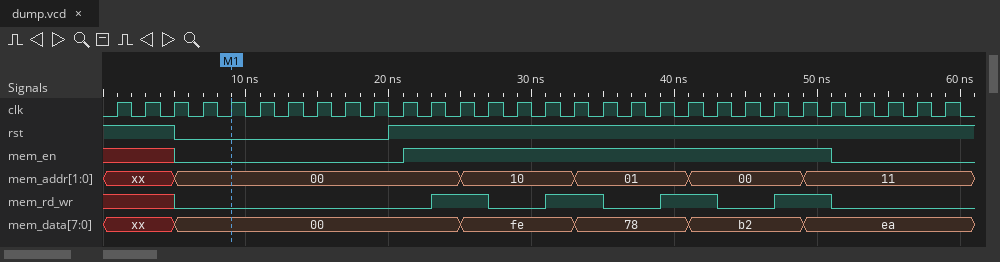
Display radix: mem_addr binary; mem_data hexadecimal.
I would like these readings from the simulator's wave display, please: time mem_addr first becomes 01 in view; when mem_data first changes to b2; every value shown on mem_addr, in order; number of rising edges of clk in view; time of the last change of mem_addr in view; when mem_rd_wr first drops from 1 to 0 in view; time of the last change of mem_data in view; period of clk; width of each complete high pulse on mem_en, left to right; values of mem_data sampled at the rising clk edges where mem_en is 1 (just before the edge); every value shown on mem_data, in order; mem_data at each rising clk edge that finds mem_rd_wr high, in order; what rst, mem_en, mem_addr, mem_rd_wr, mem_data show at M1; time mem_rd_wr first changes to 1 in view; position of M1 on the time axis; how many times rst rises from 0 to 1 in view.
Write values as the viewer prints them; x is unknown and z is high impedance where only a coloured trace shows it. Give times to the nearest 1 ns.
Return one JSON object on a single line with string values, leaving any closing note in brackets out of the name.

{"time mem_addr first becomes 01 in view": "33 ns", "when mem_data first changes to b2": "41 ns", "every value shown on mem_addr, in order": "xx, 00, 10, 01, 00, 11", "number of rising edges of clk in view": "30", "time of the last change of mem_addr in view": "49 ns", "when mem_rd_wr first drops from 1 to 0 in view": "27 ns", "time of the last change of mem_data in view": "49 ns", "period of clk": "2 ns", "width of each complete high pulse on mem_en, left to right": "30 ns", "values of mem_data sampled at the rising clk edges where mem_en is 1": "00, 00, fe, fe, fe, fe, 78, 78, 78, 78, b2, b2, b2, b2, ea", "every value shown on mem_data, in order": "xx, 00, fe, 78, b2, ea", "mem_data at each rising clk edge that finds mem_rd_wr high, in order": "00, fe, fe, 78, 78, b2, b2, ea", "what rst, mem_en, mem_addr, mem_rd_wr, mem_data show at M1": "rst=0, mem_en=0, mem_addr=00, mem_rd_wr=0, mem_data=00", "time mem_rd_wr first changes to 1 in view": "23 ns", "position of M1 on the time axis": "9 ns", "how many times rst rises from 0 to 1 in view": "1"}
